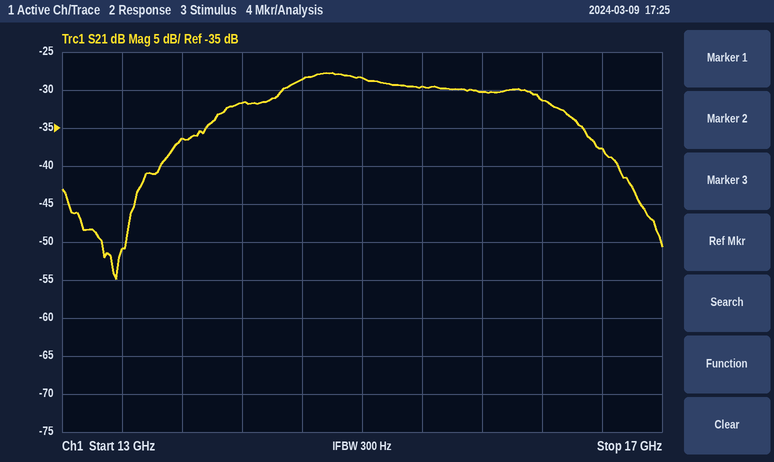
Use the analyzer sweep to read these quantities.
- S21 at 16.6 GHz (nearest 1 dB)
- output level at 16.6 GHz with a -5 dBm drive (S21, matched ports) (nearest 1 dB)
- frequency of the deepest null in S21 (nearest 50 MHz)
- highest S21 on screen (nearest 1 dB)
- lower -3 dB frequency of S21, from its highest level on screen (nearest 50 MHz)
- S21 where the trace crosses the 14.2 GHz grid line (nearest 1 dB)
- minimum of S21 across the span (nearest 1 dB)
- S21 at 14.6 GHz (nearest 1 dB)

-38 dB
-43 dBm
13.35 GHz
-28 dB
14.45 GHz
-32 dB
-55 dB
-29 dB
